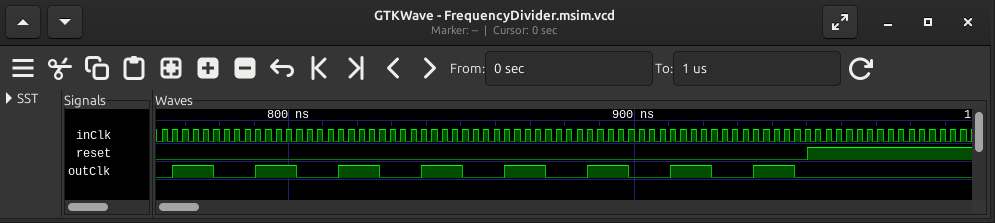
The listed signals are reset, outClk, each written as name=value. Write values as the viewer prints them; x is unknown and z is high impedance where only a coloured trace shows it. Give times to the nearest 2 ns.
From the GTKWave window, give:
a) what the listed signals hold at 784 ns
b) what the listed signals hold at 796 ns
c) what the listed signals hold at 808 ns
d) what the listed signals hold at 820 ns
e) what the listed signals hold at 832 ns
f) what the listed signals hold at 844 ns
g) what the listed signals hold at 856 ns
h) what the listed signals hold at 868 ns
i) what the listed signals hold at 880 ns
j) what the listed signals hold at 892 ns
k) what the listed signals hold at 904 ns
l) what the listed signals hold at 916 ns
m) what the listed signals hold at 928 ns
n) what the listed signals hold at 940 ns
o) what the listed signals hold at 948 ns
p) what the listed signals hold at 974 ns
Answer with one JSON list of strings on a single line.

["reset=0, outClk=0", "reset=0, outClk=1", "reset=0, outClk=0", "reset=0, outClk=1", "reset=0, outClk=0", "reset=0, outClk=1", "reset=0, outClk=0", "reset=0, outClk=1", "reset=0, outClk=0", "reset=0, outClk=1", "reset=0, outClk=0", "reset=0, outClk=1", "reset=0, outClk=0", "reset=0, outClk=1", "reset=0, outClk=0", "reset=1, outClk=0"]
